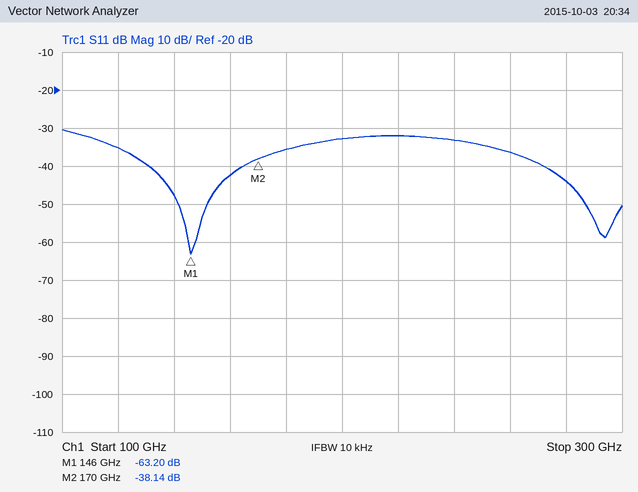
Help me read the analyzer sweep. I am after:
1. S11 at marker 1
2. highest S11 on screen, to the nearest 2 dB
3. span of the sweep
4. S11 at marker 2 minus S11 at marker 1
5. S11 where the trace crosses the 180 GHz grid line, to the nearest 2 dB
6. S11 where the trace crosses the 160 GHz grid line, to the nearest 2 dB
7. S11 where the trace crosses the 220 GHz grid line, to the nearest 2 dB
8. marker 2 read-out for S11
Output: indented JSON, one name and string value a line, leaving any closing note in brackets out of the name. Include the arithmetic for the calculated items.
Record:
{
  "S11 at marker 1": "-63.20 dB",
  "highest S11 on screen, to the nearest 2 dB": "-30 dB",
  "span of the sweep": "200 GHz",
  "S11 at marker 2 minus S11 at marker 1": "-38.14 − (-63.2) = 25.06 dB",
  "S11 where the trace crosses the 180 GHz grid line, to the nearest 2 dB": "-36 dB",
  "S11 where the trace crosses the 160 GHz grid line, to the nearest 2 dB": "-42 dB",
  "S11 where the trace crosses the 220 GHz grid line, to the nearest 2 dB": "-32 dB",
  "marker 2 read-out for S11": "-38.14 dB"
}
